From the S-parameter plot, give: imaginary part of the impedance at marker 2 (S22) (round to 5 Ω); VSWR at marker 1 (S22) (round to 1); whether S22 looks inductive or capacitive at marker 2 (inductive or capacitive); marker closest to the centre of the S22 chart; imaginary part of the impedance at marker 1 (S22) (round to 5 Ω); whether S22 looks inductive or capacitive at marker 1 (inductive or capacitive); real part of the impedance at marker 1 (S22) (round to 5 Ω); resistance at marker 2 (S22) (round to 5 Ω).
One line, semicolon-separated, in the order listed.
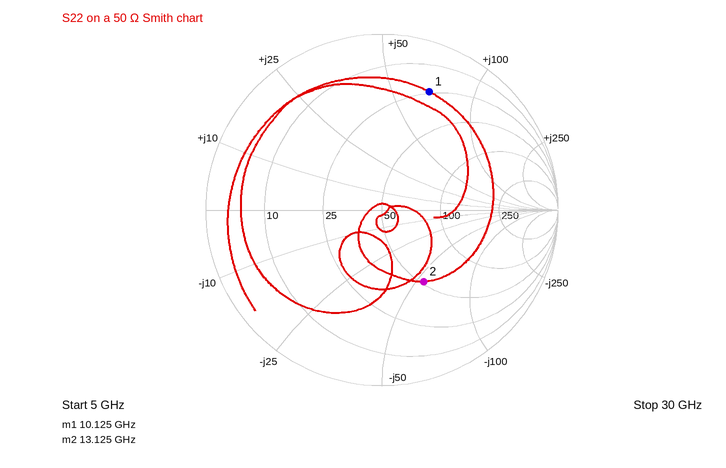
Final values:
-55 Ω; 6; capacitive; marker 2; +70 Ω; inductive; 25 Ω; 50 Ω
